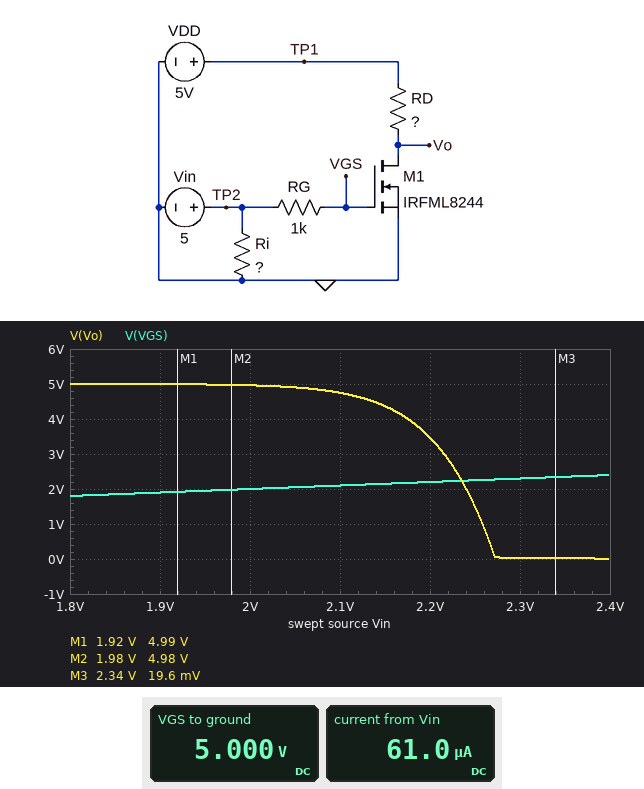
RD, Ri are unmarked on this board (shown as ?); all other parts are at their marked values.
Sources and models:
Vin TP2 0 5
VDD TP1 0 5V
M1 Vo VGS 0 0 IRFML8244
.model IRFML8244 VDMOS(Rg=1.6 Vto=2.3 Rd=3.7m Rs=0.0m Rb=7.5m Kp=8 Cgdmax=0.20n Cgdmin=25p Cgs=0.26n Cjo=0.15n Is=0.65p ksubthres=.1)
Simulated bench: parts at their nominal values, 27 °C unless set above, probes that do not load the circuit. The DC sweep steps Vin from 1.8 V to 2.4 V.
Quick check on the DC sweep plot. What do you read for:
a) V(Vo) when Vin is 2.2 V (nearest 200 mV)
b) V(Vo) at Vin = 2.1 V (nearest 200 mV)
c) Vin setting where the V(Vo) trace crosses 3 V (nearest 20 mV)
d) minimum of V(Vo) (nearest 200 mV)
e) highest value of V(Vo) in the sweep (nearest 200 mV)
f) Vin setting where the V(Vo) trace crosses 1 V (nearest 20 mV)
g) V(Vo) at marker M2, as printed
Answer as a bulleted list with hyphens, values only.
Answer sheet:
- 3.4 V
- 4.8 V
- 2.22 V
- 0 V
- 5.0 V
- 2.26 V
- 4.98 V
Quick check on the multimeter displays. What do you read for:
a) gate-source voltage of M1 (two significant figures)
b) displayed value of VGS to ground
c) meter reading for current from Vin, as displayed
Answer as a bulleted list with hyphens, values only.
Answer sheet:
- 5.0 V
- 5.000 V
- 61.0 µA
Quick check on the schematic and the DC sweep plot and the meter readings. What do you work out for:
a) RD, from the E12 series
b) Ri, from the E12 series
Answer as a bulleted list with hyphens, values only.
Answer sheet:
- 390 Ω
- 82 kΩ
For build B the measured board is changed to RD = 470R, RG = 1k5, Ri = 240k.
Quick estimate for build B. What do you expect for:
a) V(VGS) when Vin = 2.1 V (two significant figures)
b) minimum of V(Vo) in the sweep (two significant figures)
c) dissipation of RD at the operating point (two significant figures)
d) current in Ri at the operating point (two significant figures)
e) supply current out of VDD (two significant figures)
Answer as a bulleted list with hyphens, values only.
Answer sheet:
- 2.1 V
- 11 mV
- 53 mW
- 21 µA
- 11 mA
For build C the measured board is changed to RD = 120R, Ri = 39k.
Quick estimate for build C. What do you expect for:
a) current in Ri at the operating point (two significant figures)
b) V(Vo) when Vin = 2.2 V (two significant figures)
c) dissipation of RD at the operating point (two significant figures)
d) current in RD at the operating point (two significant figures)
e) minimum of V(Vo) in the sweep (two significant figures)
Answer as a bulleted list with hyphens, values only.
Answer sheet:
- 130 µA
- 4.5 V
- 210 mW
- 42 mA
- 48 mV
